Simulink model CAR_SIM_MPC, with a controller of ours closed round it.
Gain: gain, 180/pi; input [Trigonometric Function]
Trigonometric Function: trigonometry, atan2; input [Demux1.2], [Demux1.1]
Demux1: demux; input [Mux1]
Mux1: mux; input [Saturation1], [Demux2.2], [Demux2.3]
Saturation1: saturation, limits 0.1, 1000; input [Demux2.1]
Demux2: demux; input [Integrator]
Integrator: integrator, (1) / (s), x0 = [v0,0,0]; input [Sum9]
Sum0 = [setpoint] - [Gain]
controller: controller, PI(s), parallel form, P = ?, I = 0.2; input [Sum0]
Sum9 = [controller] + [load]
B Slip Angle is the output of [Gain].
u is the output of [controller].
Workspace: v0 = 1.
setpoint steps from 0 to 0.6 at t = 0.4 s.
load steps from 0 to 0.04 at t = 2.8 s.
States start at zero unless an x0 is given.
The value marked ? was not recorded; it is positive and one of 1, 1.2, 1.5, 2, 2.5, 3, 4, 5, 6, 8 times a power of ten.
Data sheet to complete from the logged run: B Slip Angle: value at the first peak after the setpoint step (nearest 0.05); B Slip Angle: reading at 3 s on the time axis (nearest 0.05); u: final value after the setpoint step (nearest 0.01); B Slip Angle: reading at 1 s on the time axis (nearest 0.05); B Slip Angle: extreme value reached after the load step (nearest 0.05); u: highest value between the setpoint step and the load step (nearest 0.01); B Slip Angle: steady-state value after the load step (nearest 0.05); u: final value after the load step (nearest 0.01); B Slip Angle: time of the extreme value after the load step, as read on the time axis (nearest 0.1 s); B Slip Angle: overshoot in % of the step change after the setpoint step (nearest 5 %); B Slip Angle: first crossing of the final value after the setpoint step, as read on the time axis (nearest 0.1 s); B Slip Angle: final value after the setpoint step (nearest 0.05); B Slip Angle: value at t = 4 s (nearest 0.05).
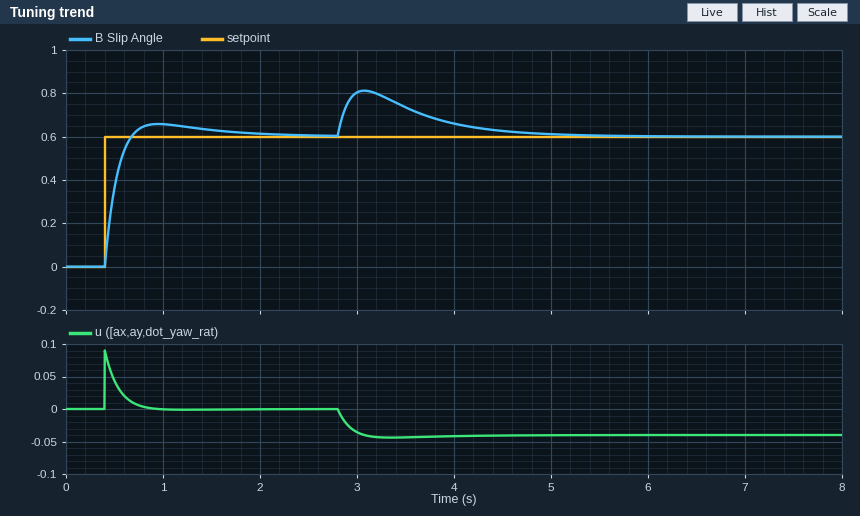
0.65
0.80
0.00
0.65
0.80
0.09
0.60
-0.04
3.1 s
10 %
0.7 s
0.60
0.65
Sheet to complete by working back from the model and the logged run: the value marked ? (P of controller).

0.15
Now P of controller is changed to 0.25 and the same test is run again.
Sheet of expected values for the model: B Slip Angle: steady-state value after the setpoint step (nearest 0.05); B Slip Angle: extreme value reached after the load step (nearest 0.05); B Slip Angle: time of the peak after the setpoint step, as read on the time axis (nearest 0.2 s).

0.60
0.75
0.8 s
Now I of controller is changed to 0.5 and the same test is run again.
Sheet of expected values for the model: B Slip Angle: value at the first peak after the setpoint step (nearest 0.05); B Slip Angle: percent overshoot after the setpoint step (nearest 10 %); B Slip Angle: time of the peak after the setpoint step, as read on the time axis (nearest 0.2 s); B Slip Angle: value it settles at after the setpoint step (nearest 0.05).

0.70
20 %
0.8 s
0.60
